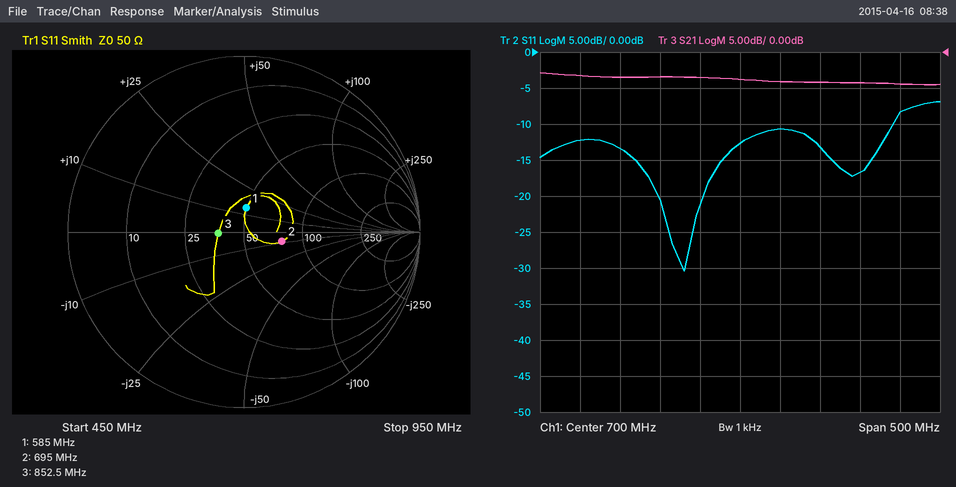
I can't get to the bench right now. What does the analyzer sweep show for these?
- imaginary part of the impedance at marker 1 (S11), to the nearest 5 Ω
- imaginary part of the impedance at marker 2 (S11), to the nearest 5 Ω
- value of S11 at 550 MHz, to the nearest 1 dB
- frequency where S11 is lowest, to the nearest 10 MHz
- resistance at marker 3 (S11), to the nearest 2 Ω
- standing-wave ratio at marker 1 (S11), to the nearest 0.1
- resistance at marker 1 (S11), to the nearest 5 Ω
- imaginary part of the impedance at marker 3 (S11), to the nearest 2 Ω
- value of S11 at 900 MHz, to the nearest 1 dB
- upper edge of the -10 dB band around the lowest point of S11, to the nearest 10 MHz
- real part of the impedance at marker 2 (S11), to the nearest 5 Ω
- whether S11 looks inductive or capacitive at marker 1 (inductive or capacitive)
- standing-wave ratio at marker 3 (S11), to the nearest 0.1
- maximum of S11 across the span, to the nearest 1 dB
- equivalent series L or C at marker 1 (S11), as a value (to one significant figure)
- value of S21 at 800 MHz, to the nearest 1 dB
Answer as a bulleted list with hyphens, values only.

- +15 Ω
- -10 Ω
- -13 dB
- 630 MHz
- 38 Ω
- 1.3
- 50 Ω
- 0 Ω
- -8 dB
- 890 MHz
- 75 Ω
- inductive
- 1.3
- -7 dB
- 4 nH
- -4 dB
